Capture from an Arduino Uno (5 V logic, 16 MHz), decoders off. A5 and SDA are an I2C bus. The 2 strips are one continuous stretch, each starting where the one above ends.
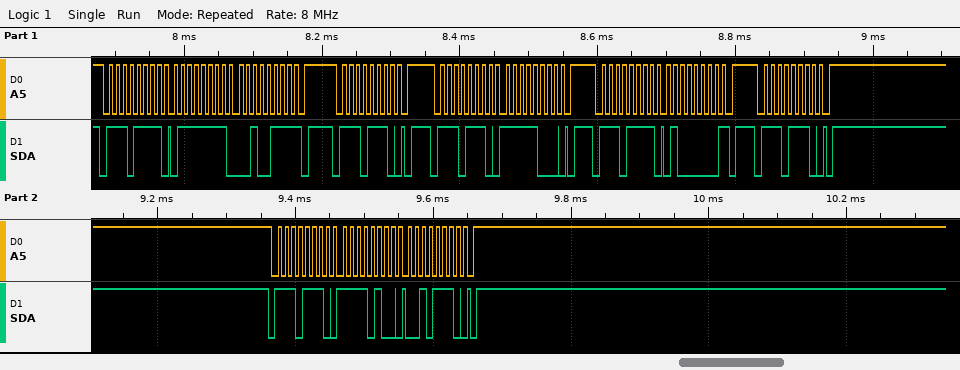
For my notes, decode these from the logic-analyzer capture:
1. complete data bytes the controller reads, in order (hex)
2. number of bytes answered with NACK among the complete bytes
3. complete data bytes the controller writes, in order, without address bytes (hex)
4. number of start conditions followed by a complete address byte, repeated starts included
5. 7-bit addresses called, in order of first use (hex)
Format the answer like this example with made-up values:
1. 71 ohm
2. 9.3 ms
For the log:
1. 7F 27 40
2. 2
3. F8 F4 2E
4. 6
5. 0x77
